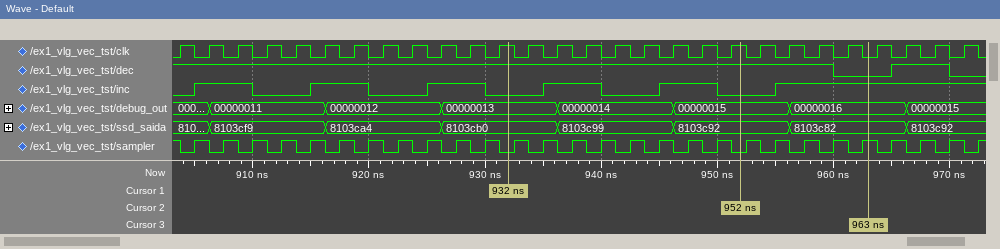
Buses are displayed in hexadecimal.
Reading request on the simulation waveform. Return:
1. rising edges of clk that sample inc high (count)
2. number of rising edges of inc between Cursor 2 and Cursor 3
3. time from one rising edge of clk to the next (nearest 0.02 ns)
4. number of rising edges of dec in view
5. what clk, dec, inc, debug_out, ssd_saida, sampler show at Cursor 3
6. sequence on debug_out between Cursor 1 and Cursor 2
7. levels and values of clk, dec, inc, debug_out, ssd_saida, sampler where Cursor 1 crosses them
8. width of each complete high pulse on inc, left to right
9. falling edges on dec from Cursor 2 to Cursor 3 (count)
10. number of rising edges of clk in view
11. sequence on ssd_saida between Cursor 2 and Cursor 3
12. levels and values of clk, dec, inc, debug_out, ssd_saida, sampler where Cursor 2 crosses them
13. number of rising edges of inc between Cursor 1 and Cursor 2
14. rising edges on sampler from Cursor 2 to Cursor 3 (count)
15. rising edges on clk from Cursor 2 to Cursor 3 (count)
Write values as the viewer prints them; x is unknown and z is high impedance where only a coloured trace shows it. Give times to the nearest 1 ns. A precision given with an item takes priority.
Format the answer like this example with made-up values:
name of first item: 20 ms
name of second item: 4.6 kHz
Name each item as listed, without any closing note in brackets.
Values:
rising edges of clk that sample inc high: 17
number of rising edges of inc between Cursor 2 and Cursor 3: 1
time from one rising edge of clk to the next: 2.5 ns
number of rising edges of dec in view: 1
what clk, dec, inc, debug_out, ssd_saida, sampler show at Cursor 3: clk=0, dec=0, inc=1, debug_out=00000016, ssd_saida=8103c82, sampler=1
sequence on debug_out between Cursor 1 and Cursor 2: 00000013, 00000014, 00000015
levels and values of clk, dec, inc, debug_out, ssd_saida, sampler where Cursor 1 crosses them: clk=1, dec=1, inc=0, debug_out=00000013, ssd_saida=8103cb0, sampler=0
width of each complete high pulse on inc, left to right: 5 ns, 5 ns, 5 ns, 5 ns, 5 ns
falling edges on dec from Cursor 2 to Cursor 3: 1
number of rising edges of clk in view: 28
sequence on ssd_saida between Cursor 2 and Cursor 3: 8103c92, 8103c82
levels and values of clk, dec, inc, debug_out, ssd_saida, sampler where Cursor 2 crosses them: clk=1, dec=1, inc=0, debug_out=00000015, ssd_saida=8103c92, sampler=0
number of rising edges of inc between Cursor 1 and Cursor 2: 2
rising edges on sampler from Cursor 2 to Cursor 3: 5
rising edges on clk from Cursor 2 to Cursor 3: 4
